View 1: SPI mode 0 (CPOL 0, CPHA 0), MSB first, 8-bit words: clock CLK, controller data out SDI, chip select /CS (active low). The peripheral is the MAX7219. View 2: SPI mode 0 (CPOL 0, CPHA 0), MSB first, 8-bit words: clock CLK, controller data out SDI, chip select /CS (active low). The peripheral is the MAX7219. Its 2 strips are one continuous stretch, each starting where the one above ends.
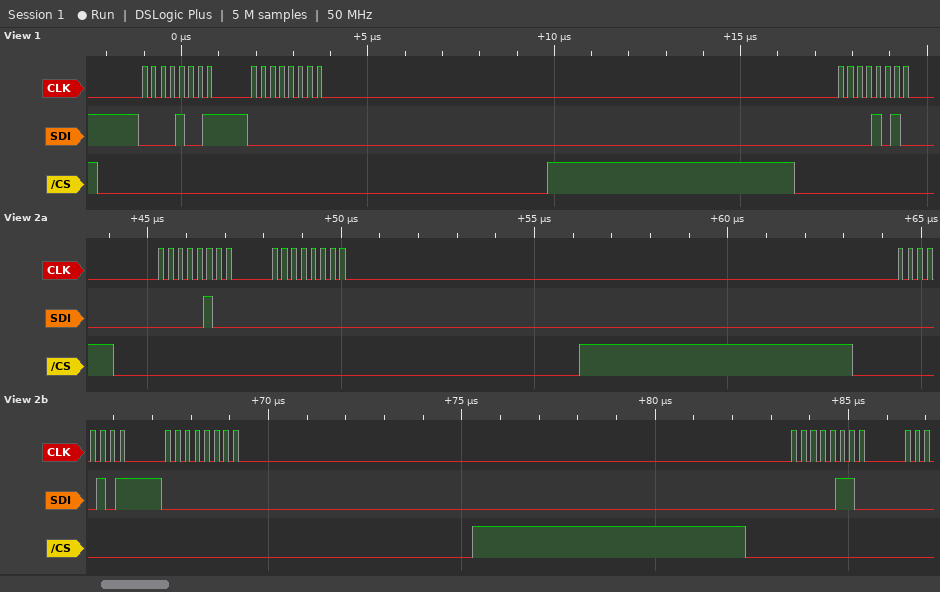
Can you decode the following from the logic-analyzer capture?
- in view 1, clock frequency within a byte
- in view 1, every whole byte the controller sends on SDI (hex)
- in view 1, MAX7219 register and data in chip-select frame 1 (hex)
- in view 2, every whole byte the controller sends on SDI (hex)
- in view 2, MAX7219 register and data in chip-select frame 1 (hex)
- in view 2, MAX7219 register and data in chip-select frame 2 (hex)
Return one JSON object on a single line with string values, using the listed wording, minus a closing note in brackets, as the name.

{"in view 1, clock frequency within a byte": "4 MHz", "in view 1, every whole byte the controller sends on SDI": "09 00 0A", "in view 1, MAX7219 register and data in chip-select frame 1": "register 0x9, data 0x00", "in view 2, every whole byte the controller sends on SDI": "04 00 05 00 06", "in view 2, MAX7219 register and data in chip-select frame 1": "register 0x4, data 0x00", "in view 2, MAX7219 register and data in chip-select frame 2": "register 0x5, data 0x00"}
